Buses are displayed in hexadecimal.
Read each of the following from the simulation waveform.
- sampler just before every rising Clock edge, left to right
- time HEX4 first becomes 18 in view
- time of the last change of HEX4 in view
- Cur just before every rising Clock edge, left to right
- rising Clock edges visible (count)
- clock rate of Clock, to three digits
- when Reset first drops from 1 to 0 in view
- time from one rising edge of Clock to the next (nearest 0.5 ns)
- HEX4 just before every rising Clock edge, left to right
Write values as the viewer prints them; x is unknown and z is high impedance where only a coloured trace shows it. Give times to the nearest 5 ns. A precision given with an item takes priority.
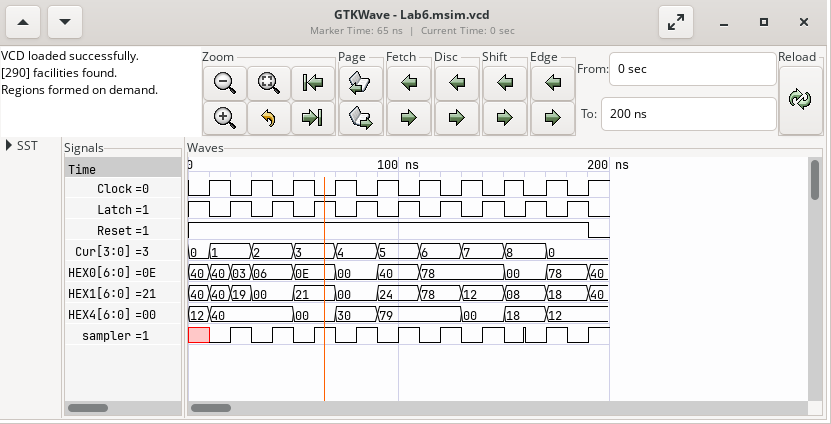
x 1 1 1 1 1 1 1 0 0
150 ns
170 ns
0, 1, 2, 3, 4, 5, 6, 7, 8, 0
10
50.0 MHz
190 ns
20 ns
12, 40, 40, 00, 30, 79, 79, 00, 18, 12
